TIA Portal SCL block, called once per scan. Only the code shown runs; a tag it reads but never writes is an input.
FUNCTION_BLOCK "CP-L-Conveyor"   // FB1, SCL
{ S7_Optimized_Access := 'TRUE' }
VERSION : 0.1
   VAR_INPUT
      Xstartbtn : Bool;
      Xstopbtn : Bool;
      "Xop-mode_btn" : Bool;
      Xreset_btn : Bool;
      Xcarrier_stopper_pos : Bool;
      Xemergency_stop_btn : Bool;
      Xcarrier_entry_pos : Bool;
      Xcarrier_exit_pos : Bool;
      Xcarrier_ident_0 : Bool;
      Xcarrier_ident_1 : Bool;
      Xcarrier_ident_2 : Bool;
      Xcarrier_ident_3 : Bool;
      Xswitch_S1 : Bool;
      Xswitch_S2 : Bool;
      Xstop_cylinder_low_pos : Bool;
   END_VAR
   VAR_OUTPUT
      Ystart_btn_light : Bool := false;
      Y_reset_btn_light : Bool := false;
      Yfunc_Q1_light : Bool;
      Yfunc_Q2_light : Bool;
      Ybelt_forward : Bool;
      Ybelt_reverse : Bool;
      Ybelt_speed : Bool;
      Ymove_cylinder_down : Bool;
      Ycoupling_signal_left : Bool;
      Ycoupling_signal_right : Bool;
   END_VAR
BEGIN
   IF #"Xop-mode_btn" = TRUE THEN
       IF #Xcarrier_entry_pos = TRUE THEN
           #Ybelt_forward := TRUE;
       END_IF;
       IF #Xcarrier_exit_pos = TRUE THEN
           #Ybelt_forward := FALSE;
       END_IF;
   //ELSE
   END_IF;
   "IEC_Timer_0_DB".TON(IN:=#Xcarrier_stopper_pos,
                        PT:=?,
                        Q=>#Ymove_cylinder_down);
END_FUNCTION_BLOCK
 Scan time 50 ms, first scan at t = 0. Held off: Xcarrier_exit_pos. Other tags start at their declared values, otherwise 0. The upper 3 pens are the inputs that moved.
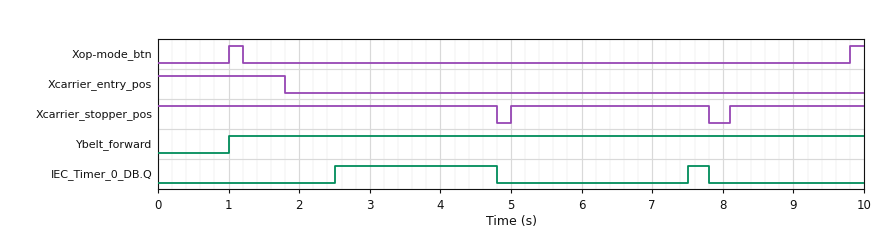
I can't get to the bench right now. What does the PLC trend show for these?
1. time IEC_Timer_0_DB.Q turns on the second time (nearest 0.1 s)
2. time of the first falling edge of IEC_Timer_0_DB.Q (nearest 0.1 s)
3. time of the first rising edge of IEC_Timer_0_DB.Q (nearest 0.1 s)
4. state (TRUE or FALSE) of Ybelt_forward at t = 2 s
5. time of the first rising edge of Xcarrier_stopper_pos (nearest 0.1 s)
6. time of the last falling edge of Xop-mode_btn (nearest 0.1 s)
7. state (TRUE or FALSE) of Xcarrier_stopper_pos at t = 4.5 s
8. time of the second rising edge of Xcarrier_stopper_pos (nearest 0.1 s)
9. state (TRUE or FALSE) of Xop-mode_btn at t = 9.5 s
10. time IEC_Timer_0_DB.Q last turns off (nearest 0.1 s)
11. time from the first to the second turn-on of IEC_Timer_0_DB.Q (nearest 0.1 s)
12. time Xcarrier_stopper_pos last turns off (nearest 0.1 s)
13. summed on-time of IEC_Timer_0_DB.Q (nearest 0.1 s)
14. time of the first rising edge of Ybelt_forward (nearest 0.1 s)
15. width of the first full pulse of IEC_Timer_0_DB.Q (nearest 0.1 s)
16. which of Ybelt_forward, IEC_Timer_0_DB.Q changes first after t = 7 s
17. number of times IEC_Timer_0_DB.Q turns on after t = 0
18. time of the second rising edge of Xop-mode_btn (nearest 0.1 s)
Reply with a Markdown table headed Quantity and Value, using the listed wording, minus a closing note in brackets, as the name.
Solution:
| Quantity | Value |
|---|---|
| time IEC_Timer_0_DB.Q turns on the second time | 7.5 s |
| time of the first falling edge of IEC_Timer_0_DB.Q | 4.8 s |
| time of the first rising edge of IEC_Timer_0_DB.Q | 2.5 s |
| state (TRUE or FALSE) of Ybelt_forward at t = 2 s | TRUE |
| time of the first rising edge of Xcarrier_stopper_pos | 5.0 s |
| time of the last falling edge of Xop-mode_btn | 1.2 s |
| state (TRUE or FALSE) of Xcarrier_stopper_pos at t = 4.5 s | TRUE |
| time of the second rising edge of Xcarrier_stopper_pos | 8.1 s |
| state (TRUE or FALSE) of Xop-mode_btn at t = 9.5 s | FALSE |
| time IEC_Timer_0_DB.Q last turns off | 7.8 s |
| time from the first to the second turn-on of IEC_Timer_0_DB.Q | 5.0 s |
| time Xcarrier_stopper_pos last turns off | 7.8 s |
| summed on-time of IEC_Timer_0_DB.Q | 2.6 s |
| time of the first rising edge of Ybelt_forward | 1.0 s |
| width of the first full pulse of IEC_Timer_0_DB.Q | 2.3 s |
| which of Ybelt_forward, IEC_Timer_0_DB.Q changes first after t = 7 s | IEC_Timer_0_DB.Q |
| number of times IEC_Timer_0_DB.Q turns on after t = 0 | 2 |
| time of the second rising edge of Xop-mode_btn | 9.8 s |
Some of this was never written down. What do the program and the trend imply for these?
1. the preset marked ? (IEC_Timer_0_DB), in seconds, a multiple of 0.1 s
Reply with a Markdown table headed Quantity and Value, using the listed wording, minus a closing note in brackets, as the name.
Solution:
| Quantity | Value |
|---|---|
| the preset marked ? (IEC_Timer_0_DB), in seconds, a multiple of 0.1 s | 2.5 s |
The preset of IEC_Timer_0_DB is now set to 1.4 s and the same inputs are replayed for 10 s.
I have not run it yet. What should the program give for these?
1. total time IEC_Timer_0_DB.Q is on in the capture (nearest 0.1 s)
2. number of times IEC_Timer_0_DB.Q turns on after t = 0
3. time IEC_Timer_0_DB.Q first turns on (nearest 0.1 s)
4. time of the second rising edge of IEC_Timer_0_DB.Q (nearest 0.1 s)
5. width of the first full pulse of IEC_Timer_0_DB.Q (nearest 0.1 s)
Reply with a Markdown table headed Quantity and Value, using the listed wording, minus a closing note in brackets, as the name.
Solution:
| Quantity | Value |
|---|---|
| total time IEC_Timer_0_DB.Q is on in the capture | 5.3 s |
| number of times IEC_Timer_0_DB.Q turns on after t = 0 | 3 |
| time IEC_Timer_0_DB.Q first turns on | 1.4 s |
| time of the second rising edge of IEC_Timer_0_DB.Q | 6.4 s |
| width of the first full pulse of IEC_Timer_0_DB.Q | 3.4 s |
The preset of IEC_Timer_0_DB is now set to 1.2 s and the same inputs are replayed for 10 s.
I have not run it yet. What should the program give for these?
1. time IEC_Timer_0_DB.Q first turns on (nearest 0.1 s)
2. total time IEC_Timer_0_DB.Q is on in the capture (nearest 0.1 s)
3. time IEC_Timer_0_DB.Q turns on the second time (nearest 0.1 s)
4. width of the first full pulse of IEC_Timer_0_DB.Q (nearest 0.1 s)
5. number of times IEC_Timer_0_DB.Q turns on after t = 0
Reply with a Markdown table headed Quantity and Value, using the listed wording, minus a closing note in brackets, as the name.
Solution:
| Quantity | Value |
|---|---|
| time IEC_Timer_0_DB.Q first turns on | 1.2 s |
| total time IEC_Timer_0_DB.Q is on in the capture | 5.9 s |
| time IEC_Timer_0_DB.Q turns on the second time | 6.2 s |
| width of the first full pulse of IEC_Timer_0_DB.Q | 3.6 s |
| number of times IEC_Timer_0_DB.Q turns on after t = 0 | 3 |
